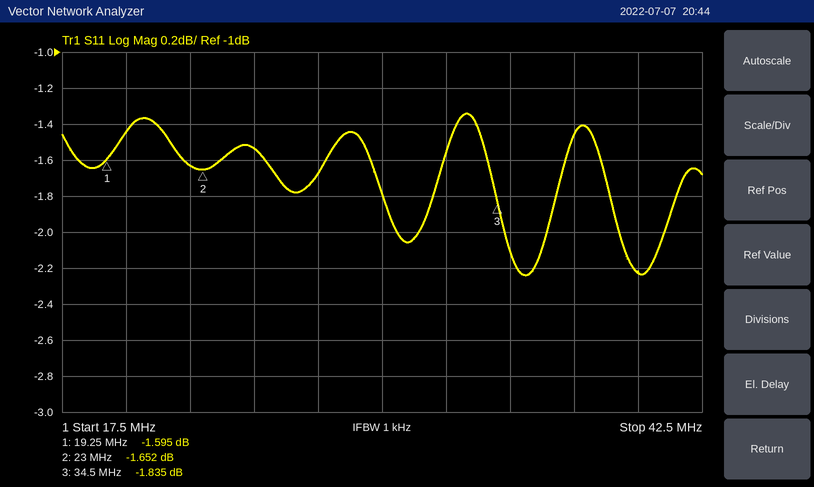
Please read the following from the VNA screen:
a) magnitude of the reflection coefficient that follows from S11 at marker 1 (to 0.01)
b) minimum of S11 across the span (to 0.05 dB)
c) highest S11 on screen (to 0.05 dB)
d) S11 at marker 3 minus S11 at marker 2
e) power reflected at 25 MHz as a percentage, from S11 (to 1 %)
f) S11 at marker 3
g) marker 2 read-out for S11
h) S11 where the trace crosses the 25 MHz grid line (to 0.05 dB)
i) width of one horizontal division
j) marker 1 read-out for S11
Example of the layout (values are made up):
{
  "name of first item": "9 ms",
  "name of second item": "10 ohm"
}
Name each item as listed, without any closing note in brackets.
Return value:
{
  "magnitude of the reflection coefficient that follows from S11 at marker 1": "0.83",
  "minimum of S11 across the span": "-2.25 dB",
  "highest S11 on screen": "-1.35 dB",
  "S11 at marker 3 minus S11 at marker 2": "-0.183 dB",
  "power reflected at 25 MHz as a percentage, from S11": "70 %",
  "S11 at marker 3": "-1.835 dB",
  "marker 2 read-out for S11": "-1.652 dB",
  "S11 where the trace crosses the 25 MHz grid line": "-1.55 dB",
  "width of one horizontal division": "2.5 MHz",
  "marker 1 read-out for S11": "-1.595 dB"
}
